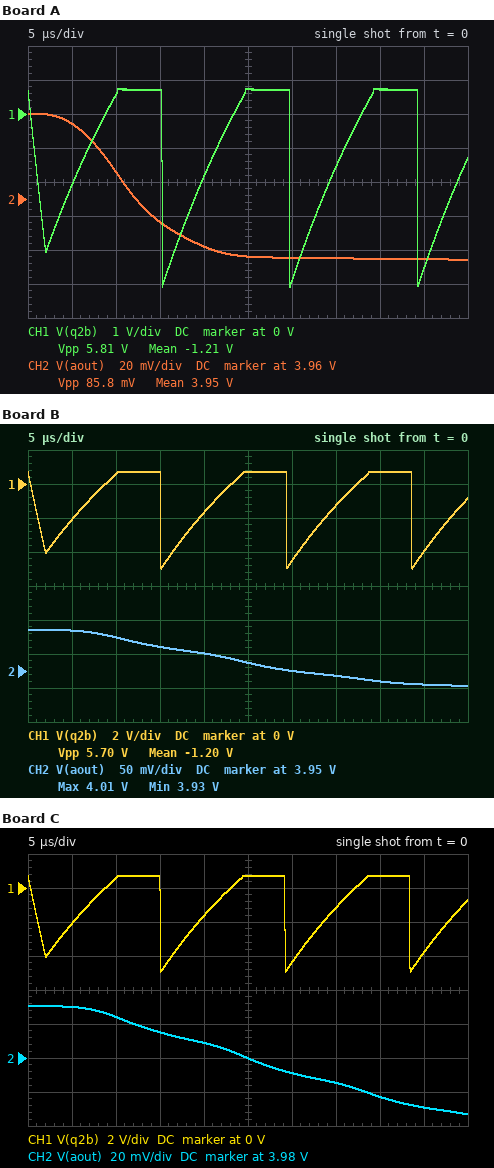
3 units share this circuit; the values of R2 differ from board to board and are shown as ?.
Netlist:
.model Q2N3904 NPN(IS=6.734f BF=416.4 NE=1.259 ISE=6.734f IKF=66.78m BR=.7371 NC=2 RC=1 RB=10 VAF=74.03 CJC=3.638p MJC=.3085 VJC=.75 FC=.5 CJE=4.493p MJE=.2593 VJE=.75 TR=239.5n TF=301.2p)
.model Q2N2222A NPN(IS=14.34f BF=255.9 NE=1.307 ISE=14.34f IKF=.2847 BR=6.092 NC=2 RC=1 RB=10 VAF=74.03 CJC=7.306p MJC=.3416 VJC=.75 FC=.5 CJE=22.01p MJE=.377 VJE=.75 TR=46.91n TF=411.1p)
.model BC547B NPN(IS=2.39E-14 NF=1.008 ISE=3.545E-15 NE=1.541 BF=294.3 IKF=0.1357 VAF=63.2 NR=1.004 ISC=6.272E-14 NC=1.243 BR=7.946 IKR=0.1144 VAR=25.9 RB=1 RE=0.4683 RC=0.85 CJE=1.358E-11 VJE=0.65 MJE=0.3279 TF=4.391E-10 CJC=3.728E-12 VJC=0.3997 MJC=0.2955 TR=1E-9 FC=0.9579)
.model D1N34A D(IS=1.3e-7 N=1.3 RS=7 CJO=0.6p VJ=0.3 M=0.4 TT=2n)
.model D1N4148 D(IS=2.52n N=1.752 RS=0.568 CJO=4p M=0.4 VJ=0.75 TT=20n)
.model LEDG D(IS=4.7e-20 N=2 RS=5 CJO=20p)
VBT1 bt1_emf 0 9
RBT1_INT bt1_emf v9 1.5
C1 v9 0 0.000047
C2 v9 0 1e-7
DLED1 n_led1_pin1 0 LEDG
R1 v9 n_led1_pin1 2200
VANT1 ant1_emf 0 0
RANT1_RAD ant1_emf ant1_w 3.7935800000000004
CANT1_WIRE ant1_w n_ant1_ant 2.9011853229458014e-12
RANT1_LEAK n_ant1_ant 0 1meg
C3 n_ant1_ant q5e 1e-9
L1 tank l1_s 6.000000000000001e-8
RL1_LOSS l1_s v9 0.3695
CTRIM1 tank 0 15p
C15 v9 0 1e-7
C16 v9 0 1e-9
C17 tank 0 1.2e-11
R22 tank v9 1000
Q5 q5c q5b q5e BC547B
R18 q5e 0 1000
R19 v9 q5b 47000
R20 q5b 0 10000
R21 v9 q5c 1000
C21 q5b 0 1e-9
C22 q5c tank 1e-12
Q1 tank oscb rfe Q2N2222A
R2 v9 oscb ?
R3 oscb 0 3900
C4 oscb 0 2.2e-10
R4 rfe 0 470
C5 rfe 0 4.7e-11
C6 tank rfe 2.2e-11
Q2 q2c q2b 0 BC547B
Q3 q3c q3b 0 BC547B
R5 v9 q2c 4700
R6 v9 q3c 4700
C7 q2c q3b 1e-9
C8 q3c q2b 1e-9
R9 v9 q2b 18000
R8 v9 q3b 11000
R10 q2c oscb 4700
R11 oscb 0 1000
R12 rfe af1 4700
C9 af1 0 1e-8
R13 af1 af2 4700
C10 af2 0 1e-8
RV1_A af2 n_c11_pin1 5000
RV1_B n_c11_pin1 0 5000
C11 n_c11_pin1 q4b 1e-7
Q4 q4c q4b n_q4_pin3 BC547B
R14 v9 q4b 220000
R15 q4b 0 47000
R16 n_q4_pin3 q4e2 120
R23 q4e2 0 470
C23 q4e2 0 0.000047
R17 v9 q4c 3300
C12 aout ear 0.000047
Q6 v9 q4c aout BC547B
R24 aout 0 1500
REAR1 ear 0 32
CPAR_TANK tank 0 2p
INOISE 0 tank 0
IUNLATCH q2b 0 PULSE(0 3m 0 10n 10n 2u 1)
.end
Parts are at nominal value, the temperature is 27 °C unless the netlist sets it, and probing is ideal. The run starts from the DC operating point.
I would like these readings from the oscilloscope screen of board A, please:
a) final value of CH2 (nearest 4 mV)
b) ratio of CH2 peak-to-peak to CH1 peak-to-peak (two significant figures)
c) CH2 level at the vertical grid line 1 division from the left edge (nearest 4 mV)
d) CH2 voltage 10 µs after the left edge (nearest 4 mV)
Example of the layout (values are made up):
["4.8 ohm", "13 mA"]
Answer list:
["3.924 V", "0.015", "4.004 V", "3.976 V"]
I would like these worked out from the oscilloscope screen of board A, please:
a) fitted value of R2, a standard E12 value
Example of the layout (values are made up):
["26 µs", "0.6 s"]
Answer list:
["10 kΩ"]
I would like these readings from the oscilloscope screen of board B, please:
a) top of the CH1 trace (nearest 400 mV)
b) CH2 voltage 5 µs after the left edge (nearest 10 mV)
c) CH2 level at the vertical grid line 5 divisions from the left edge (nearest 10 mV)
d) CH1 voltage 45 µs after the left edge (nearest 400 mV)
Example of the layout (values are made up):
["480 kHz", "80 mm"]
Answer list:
["800 mV", "4.01 V", "3.96 V", "-4.0 V"]
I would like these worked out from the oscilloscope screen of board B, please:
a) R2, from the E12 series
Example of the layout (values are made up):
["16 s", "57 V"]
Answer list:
["27 kΩ"]
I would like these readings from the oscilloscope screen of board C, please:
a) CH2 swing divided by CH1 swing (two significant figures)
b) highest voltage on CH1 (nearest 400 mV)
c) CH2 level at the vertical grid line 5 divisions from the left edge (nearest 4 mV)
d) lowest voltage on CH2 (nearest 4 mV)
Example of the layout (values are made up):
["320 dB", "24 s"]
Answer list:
["0.011", "800 mV", "3.980 V", "3.948 V"]
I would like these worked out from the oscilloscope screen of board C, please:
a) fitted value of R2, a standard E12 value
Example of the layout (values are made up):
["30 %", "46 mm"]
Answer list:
["47 kΩ"]
